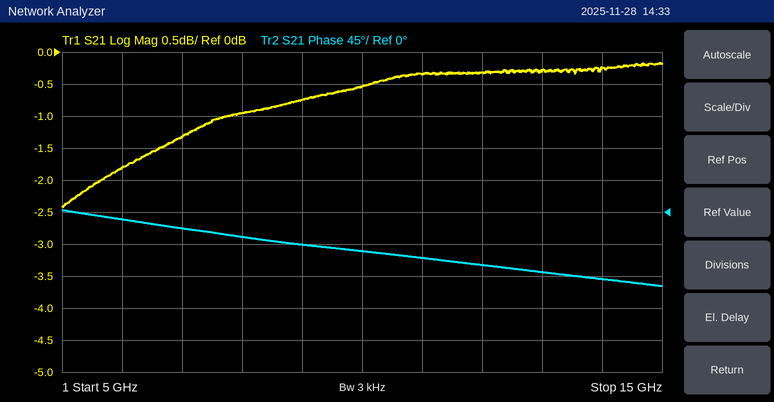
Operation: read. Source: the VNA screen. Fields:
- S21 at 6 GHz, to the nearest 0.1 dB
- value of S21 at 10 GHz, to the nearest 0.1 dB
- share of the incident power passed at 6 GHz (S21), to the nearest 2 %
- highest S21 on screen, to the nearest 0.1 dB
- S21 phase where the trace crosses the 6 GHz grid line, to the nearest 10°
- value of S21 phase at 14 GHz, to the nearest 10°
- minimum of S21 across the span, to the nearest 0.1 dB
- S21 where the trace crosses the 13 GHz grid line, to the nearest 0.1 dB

-1.8 dB
-0.5 dB
66 %
-0.2 dB
-10°
-90°
-2.4 dB
-0.3 dB
